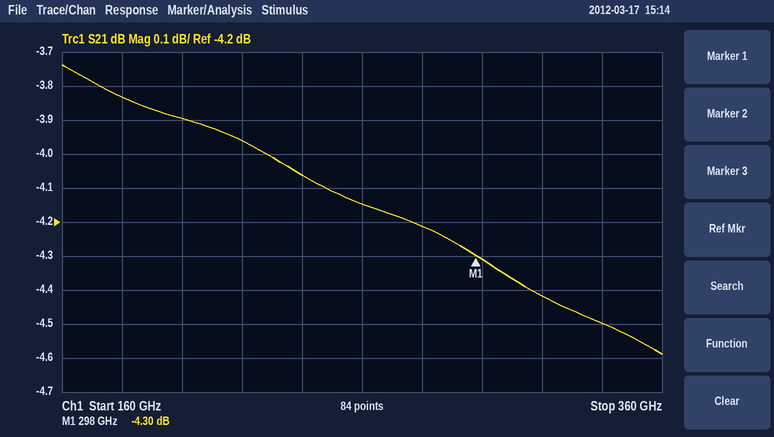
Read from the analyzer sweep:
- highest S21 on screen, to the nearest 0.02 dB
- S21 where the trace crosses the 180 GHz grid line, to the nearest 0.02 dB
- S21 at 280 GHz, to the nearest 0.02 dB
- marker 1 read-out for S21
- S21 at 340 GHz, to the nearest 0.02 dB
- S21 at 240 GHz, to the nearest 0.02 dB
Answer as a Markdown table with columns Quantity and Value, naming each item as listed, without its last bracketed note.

| Quantity | Value |
|---|---|
| highest S21 on screen, to the nearest 0.02 dB | -3.74 dB |
| S21 where the trace crosses the 180 GHz grid line, to the nearest 0.02 dB | -3.84 dB |
| S21 at 280 GHz, to the nearest 0.02 dB | -4.22 dB |
| marker 1 read-out for S21 | -4.30 dB |
| S21 at 340 GHz, to the nearest 0.02 dB | -4.50 dB |
| S21 at 240 GHz, to the nearest 0.02 dB | -4.06 dB |
